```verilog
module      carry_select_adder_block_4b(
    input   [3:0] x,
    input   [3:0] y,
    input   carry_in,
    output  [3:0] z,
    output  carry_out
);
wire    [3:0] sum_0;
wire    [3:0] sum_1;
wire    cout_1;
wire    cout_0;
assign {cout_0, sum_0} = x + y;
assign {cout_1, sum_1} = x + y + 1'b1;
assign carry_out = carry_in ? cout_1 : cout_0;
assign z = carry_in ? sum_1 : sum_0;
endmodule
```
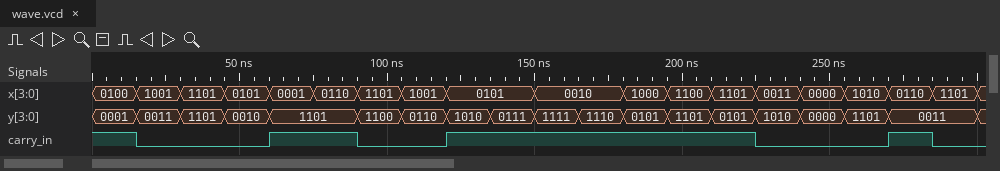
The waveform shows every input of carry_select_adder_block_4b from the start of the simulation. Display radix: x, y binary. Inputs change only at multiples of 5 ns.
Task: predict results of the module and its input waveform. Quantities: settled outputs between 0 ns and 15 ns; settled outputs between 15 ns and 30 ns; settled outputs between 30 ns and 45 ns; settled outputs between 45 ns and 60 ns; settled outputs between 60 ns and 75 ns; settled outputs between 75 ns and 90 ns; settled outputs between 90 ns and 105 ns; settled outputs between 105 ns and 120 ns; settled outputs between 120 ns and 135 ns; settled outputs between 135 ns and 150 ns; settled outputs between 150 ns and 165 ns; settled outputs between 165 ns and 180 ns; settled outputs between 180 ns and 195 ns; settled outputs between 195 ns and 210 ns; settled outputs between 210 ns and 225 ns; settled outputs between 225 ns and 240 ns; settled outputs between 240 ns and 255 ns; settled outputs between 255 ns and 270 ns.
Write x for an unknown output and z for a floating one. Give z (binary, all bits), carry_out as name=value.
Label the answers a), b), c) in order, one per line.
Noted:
a) z=0110, carry_out=0
b) z=1100, carry_out=0
c) z=1010, carry_out=1
d) z=0111, carry_out=0
e) z=1111, carry_out=0
f) z=0100, carry_out=1
g) z=1001, carry_out=1
h) z=1111, carry_out=0
i) z=0000, carry_out=1
j) z=1101, carry_out=0
k) z=0010, carry_out=1
l) z=0001, carry_out=1
m) z=1110, carry_out=0
n) z=1010, carry_out=1
o) z=0011, carry_out=1
p) z=1101, carry_out=0
q) z=0000, carry_out=0
r) z=0111, carry_out=1
